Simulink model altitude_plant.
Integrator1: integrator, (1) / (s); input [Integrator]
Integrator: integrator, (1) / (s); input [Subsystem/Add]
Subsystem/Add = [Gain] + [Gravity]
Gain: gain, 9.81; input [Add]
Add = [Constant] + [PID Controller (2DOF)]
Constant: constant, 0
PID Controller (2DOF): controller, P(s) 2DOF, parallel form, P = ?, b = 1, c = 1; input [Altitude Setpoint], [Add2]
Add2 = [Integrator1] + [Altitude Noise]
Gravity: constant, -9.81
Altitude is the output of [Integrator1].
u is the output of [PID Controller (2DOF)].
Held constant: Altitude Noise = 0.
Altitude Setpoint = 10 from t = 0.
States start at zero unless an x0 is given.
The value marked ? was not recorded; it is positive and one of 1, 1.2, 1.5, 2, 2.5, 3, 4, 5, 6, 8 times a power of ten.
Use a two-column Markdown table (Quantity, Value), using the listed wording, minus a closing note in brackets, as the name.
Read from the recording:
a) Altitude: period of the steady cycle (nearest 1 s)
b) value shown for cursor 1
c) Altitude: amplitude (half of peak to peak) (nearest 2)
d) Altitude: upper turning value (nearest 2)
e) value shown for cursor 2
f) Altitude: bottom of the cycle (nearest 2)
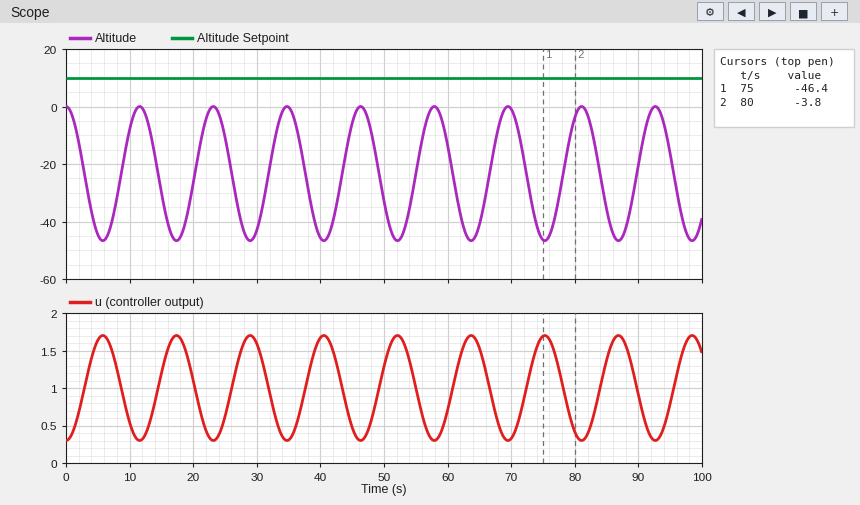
| Quantity | Value |
|---|---|
| Altitude: period of the steady cycle | 12 s |
| value shown for cursor 1 | -46.4 |
| Altitude: amplitude (half of peak to peak) | 24 |
| Altitude: upper turning value | 0 |
| value shown for cursor 2 | -3.8 |
| Altitude: bottom of the cycle | -46 |
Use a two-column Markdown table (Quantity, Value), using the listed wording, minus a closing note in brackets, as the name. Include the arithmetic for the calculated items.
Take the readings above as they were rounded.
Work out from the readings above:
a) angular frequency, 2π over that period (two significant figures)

| Quantity | Value |
|---|---|
| angular frequency, 2π over that period | 2π / 12 = 0.52 rad/s |
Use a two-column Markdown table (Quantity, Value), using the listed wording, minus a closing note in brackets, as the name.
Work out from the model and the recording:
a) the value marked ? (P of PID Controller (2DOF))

| Quantity | Value |
|---|---|
| the value marked ? (P of PID Controller (2DOF)) | 0.03 |
